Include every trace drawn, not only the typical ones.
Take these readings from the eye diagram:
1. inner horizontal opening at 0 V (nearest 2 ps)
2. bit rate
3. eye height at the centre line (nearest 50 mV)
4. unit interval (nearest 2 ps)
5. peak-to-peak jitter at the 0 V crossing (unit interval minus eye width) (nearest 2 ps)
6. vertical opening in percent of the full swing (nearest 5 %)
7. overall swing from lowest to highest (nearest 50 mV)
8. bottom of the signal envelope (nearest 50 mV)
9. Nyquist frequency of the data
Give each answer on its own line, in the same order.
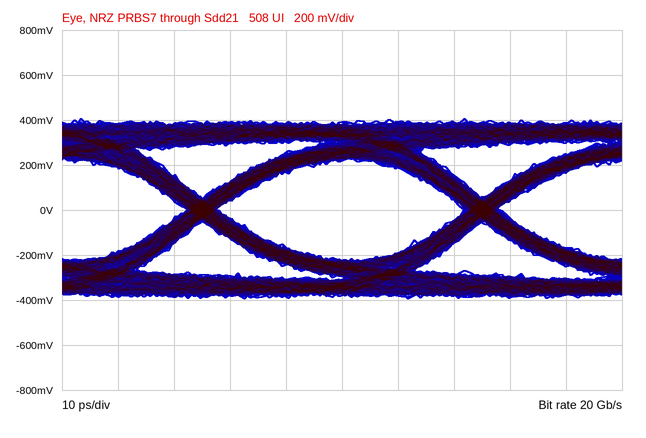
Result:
44 ps
20 Gb/s
450 mV
50 ps
6 ps
55 %
800 mV
-400 mV
10 GHz
